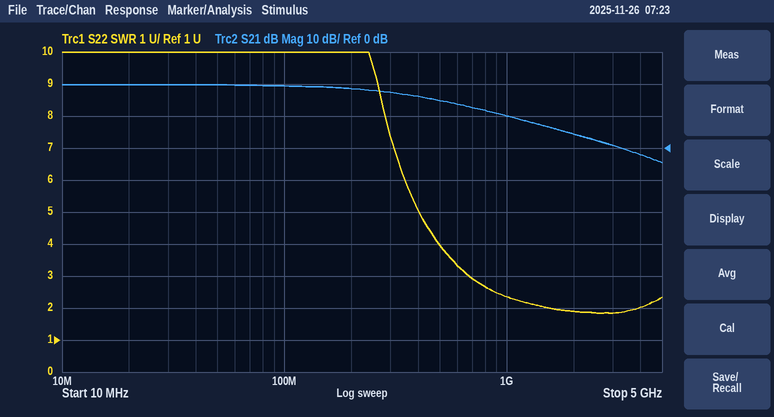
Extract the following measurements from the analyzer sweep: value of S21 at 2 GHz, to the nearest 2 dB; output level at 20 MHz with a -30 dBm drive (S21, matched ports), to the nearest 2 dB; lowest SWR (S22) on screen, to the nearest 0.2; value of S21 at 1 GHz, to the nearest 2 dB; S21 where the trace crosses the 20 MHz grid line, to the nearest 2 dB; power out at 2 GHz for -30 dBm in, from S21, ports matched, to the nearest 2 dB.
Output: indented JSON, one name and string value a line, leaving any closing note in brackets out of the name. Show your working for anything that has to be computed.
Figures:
{
  "value of S21 at 2 GHz, to the nearest 2 dB": "4 dB",
  "output level at 20 MHz with a -30 dBm drive (S21, matched ports), to the nearest 2 dB": "-30 dBm + (20 dB) = -10 dBm",
  "lowest SWR (S22) on screen, to the nearest 0.2": "1.8",
  "value of S21 at 1 GHz, to the nearest 2 dB": "10 dB",
  "S21 where the trace crosses the 20 MHz grid line, to the nearest 2 dB": "20 dB",
  "power out at 2 GHz for -30 dBm in, from S21, ports matched, to the nearest 2 dB": "-30 dBm + (4 dB) = -26 dBm"
}
